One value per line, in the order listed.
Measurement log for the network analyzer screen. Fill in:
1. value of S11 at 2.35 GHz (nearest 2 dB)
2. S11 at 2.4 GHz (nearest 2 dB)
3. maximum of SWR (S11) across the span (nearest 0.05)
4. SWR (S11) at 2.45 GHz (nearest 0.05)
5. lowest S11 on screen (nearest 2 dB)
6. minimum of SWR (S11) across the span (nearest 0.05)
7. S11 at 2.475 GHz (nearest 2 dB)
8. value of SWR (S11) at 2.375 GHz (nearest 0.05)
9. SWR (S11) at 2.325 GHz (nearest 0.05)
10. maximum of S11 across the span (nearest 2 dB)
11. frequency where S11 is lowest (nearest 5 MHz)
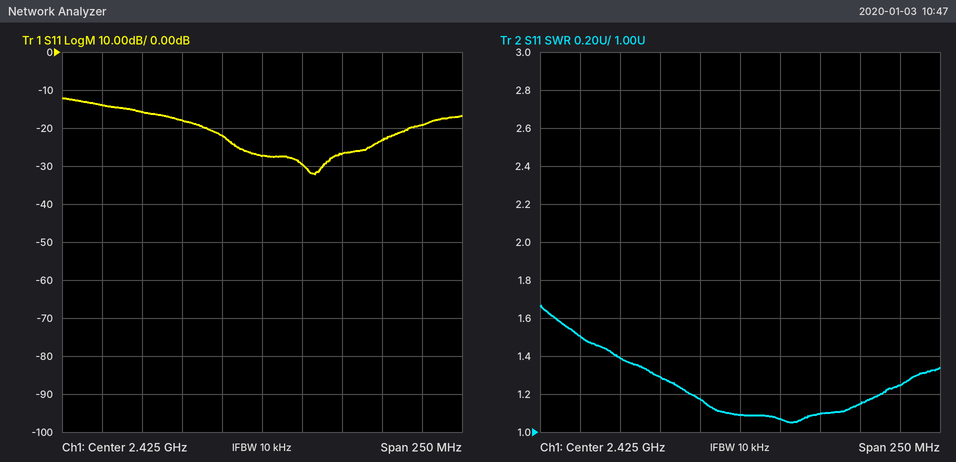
-16 dB
-22 dB
1.65
1.05
-32 dB
1.05
-26 dB
1.30
1.50
-12 dB
2.460 GHz
